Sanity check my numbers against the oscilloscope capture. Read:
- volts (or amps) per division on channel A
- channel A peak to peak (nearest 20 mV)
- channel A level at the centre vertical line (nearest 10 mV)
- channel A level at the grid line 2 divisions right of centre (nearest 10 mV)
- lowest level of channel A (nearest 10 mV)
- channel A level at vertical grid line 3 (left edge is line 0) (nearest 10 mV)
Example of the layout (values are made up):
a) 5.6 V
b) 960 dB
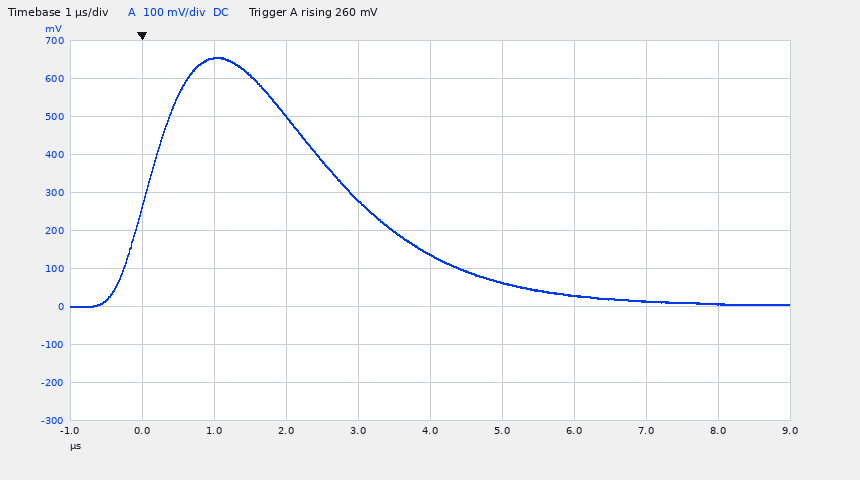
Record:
a) 100 mV
b) 660 mV
c) 140 mV
d) 30 mV
e) 0 mV
f) 500 mV
